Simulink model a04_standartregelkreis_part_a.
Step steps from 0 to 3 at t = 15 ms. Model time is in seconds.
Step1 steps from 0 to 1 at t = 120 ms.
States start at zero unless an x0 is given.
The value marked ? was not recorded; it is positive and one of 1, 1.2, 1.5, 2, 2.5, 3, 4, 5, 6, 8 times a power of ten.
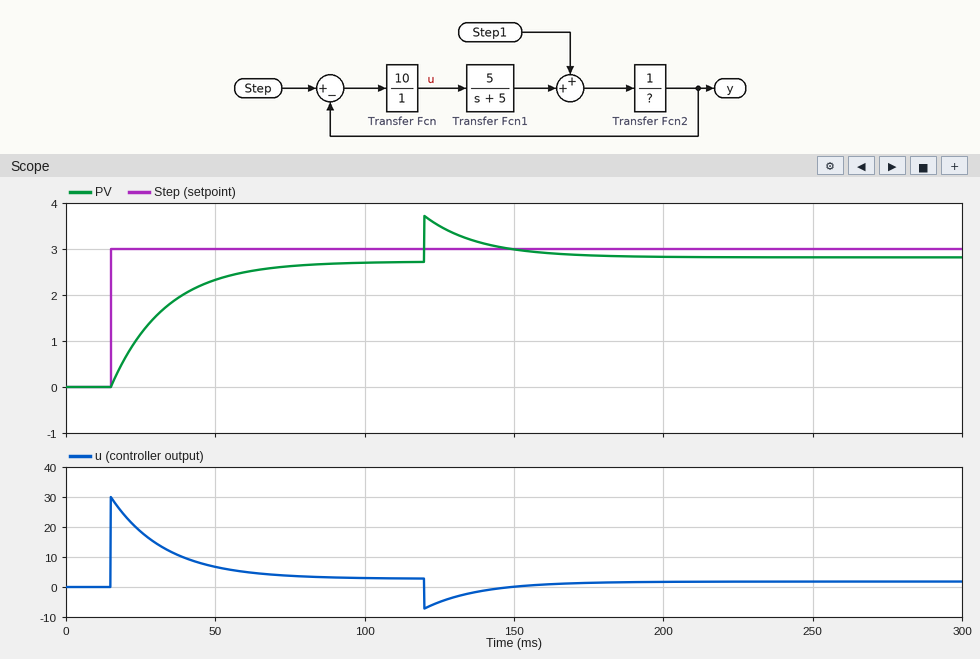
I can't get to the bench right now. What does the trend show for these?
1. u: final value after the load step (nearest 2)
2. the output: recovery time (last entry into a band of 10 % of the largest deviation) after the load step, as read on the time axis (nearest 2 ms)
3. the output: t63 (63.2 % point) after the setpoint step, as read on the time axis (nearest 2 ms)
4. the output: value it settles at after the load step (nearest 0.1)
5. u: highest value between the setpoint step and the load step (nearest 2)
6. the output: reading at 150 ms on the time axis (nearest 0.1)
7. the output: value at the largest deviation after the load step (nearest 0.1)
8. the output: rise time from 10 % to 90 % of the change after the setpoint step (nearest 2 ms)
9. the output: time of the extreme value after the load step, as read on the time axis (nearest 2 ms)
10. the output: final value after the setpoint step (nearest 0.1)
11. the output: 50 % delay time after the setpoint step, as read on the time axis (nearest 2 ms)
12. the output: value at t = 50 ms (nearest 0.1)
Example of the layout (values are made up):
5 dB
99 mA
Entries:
2
160 ms
34 ms
2.8
30
3.0
3.7
40 ms
120 ms
2.7
28 ms
2.3
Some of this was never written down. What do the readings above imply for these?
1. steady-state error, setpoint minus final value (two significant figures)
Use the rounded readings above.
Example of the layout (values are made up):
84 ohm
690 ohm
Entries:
0.30
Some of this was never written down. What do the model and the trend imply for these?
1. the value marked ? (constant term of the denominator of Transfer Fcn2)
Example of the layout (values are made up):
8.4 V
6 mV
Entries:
1
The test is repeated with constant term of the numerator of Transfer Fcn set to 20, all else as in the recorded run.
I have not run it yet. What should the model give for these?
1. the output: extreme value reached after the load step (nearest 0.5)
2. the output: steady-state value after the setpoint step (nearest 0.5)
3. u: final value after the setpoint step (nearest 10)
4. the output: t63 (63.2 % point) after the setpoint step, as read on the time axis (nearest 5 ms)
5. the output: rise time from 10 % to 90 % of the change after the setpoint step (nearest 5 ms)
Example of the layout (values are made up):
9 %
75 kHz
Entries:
4.0
3.0
0
25 ms
20 ms
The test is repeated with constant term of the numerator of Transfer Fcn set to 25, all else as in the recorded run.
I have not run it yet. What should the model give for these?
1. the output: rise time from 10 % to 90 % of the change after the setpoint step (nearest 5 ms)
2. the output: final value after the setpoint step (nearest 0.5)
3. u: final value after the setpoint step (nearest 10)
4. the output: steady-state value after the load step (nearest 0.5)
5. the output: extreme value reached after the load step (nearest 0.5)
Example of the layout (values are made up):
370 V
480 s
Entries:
15 ms
3.0
0
3.0
4.0
